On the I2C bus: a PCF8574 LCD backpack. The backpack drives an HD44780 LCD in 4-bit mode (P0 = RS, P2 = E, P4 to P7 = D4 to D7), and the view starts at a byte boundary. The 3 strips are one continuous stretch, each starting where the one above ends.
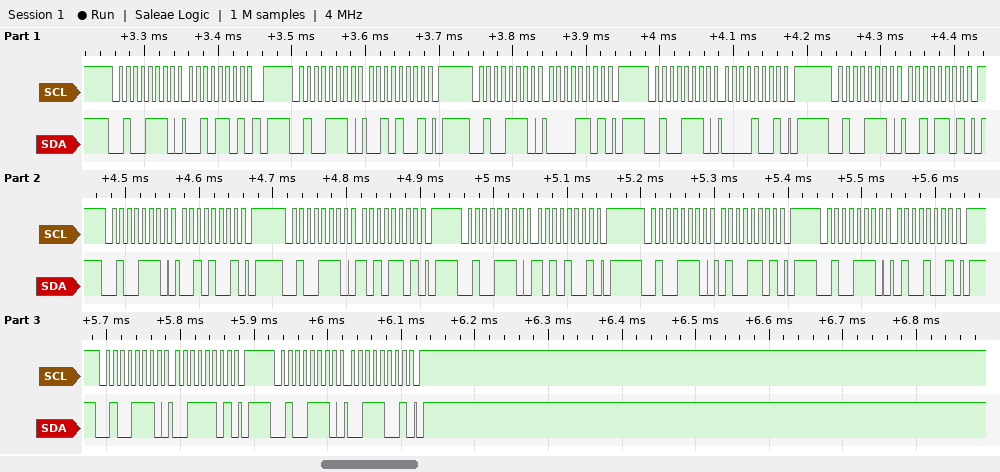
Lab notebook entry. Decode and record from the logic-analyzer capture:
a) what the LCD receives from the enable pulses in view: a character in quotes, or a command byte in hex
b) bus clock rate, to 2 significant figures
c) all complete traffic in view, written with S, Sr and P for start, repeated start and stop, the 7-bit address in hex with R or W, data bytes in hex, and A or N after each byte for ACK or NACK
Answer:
' ' '*' 'C'
100 kHz
S 27W A 2D A P S 27W A 29 A P S 27W A 0D A P S 27W A 09 A P S 27W A 2D A P S 27W A 29 A P S 27W A AD A P S 27W A A9 A P S 27W A 4D A P S 27W A 49 A P S 27W A 3D A P S 27W A 39 A P
